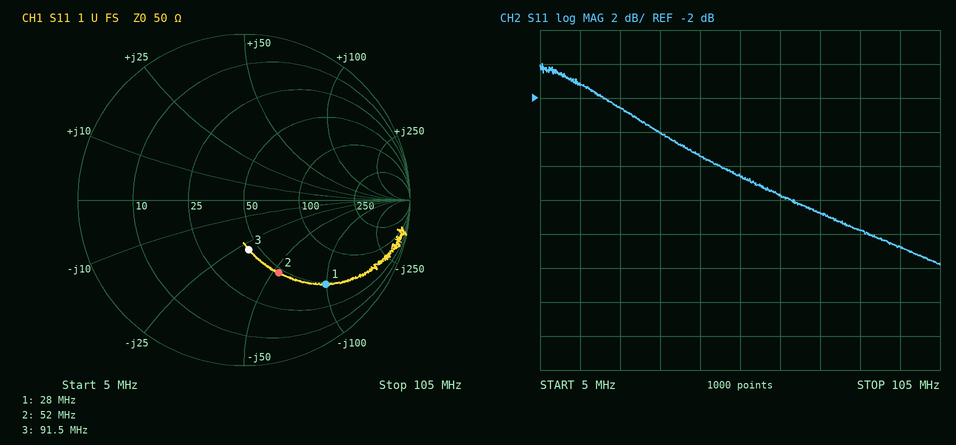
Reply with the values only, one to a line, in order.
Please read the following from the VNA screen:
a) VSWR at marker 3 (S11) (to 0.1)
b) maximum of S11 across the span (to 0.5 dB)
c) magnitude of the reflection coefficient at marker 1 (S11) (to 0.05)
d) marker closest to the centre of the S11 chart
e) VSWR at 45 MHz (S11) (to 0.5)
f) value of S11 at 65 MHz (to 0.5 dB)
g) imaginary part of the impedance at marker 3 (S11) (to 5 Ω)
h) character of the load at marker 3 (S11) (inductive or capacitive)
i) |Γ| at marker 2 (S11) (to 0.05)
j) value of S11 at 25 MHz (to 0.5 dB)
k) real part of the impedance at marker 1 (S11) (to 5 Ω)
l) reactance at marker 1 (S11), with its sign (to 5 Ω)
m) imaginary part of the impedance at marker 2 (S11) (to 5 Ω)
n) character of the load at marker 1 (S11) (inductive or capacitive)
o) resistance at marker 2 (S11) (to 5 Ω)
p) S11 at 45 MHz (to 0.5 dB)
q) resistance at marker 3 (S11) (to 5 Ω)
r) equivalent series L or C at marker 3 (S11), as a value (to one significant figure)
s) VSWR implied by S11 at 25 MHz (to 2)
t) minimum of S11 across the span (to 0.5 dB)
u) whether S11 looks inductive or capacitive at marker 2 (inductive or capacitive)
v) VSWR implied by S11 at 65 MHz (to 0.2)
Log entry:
1.9
0.0 dB
0.70
marker 3
3.5
-7.5 dB
-30 Ω
capacitive
0.50
-2.5 dB
50 Ω
-100 Ω
-55 Ω
capacitive
45 Ω
-5.5 dB
45 Ω
60 pF
6
-12.0 dB
capacitive
2.4
